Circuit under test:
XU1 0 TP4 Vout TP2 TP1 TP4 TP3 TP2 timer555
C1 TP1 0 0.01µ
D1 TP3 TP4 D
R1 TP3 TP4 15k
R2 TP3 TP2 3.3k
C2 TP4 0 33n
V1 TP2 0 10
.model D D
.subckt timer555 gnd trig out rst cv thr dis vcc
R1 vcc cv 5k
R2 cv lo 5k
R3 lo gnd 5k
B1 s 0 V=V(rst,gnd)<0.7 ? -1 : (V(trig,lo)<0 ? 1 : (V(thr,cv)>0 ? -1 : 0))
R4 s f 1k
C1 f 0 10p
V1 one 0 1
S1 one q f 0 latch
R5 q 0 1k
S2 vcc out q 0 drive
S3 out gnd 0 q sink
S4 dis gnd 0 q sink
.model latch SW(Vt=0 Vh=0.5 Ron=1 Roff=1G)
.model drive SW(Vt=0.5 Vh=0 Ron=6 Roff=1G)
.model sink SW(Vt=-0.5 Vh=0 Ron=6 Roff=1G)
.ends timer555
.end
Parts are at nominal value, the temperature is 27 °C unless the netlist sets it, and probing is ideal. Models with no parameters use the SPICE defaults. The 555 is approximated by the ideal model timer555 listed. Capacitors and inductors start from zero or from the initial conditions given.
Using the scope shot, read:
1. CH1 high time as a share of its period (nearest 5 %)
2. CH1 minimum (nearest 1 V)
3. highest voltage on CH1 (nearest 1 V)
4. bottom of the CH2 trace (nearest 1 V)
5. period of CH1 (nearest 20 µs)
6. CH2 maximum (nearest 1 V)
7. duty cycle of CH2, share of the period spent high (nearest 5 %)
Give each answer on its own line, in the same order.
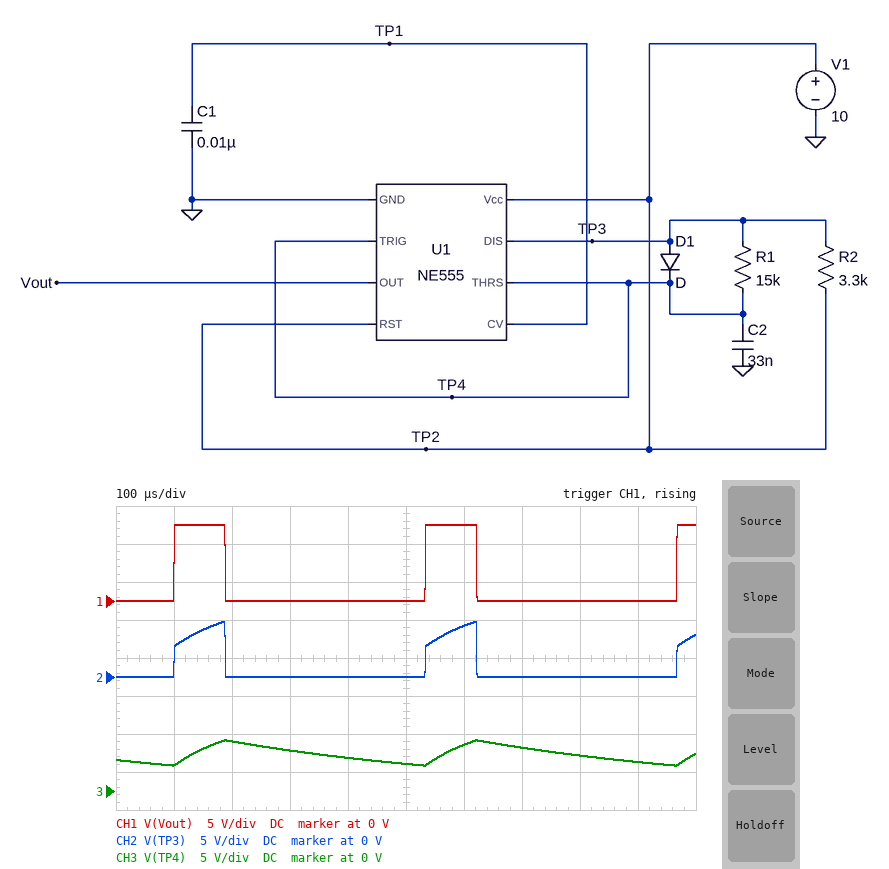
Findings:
20 %
0 V
10 V
0 V
440 µs
7 V
20 %
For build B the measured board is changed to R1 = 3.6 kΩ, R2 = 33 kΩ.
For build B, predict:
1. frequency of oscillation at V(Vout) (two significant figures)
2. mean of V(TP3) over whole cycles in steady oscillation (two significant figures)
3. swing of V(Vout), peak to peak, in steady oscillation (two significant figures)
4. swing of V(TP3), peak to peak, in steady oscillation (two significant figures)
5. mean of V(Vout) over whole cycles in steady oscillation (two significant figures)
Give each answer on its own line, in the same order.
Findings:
1.1 kHz
5.1 V
10 V
7.0 V
9.1 V
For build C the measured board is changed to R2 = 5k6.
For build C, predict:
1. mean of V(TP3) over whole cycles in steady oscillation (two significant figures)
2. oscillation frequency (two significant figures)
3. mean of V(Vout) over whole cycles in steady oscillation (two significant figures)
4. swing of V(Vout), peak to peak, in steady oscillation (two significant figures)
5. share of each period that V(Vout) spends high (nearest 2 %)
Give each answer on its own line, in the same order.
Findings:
1.8 V
2.0 kHz
3.0 V
10 V
30 %
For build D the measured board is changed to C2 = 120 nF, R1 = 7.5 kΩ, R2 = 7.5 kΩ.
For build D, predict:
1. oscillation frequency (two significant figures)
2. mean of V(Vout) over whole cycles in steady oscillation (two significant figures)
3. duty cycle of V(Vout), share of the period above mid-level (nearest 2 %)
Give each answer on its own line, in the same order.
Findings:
740 Hz
5.4 V
54 %
